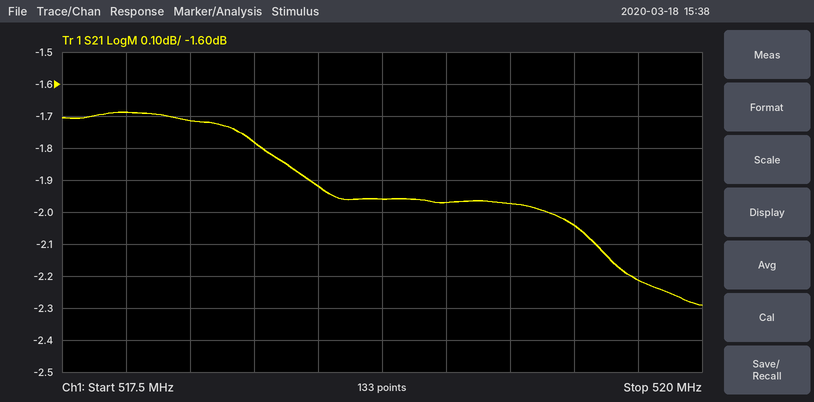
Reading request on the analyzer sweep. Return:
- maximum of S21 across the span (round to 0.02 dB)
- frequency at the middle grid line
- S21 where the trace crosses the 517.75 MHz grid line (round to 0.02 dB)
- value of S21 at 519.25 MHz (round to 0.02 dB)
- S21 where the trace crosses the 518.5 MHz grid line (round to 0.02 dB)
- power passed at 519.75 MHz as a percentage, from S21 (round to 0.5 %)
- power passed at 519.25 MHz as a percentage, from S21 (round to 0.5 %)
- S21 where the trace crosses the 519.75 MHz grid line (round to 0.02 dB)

-1.68 dB
518.75 MHz
-1.68 dB
-1.98 dB
-1.92 dB
60.0 %
63.5 %
-2.22 dB
